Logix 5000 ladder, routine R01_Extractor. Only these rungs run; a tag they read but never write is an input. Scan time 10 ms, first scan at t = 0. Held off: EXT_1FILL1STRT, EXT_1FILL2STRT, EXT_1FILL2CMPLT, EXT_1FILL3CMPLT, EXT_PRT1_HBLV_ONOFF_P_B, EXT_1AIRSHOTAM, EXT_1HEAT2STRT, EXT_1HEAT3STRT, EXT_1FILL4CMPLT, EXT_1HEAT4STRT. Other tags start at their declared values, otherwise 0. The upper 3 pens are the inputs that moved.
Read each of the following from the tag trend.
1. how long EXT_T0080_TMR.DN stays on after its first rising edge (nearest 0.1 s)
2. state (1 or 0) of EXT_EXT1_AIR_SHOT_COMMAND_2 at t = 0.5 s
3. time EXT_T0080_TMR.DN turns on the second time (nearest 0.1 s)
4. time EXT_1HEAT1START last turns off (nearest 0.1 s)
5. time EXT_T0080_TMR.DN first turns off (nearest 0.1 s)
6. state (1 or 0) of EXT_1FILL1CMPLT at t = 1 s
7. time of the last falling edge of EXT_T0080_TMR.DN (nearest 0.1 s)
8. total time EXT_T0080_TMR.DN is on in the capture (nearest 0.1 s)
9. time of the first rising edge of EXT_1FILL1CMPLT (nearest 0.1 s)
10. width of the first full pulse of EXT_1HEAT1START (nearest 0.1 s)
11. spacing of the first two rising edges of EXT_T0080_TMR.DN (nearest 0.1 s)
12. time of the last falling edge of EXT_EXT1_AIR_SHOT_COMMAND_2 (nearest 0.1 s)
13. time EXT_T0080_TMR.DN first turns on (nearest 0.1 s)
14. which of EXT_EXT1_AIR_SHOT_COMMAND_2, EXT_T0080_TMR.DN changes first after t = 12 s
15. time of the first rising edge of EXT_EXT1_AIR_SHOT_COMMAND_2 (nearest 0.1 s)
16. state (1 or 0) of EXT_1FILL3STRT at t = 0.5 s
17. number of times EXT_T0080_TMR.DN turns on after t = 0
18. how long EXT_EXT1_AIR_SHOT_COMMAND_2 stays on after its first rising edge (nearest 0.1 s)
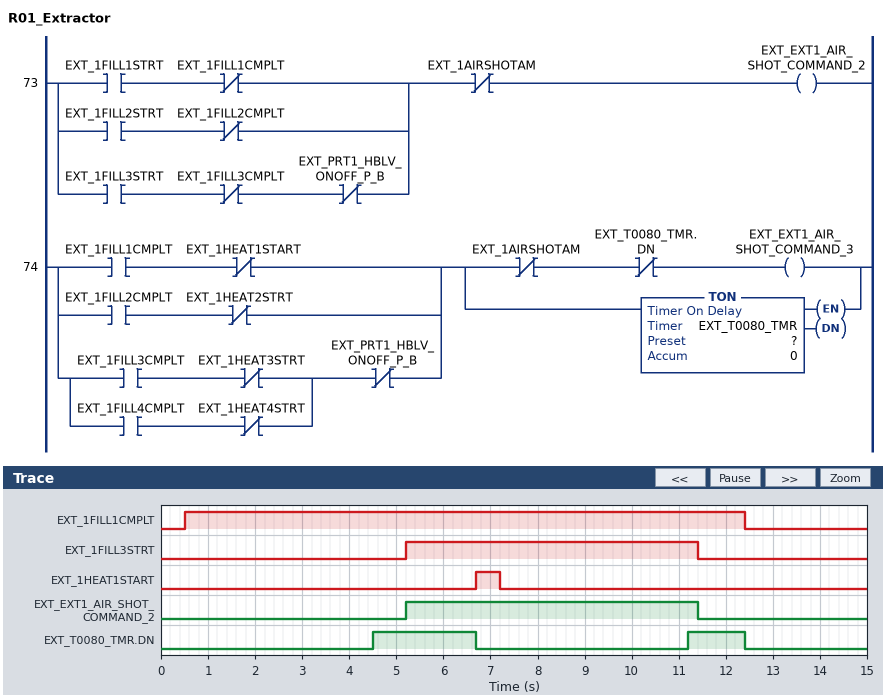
2.2 s
0
11.2 s
7.2 s
6.7 s
1
12.4 s
3.4 s
0.5 s
0.5 s
6.7 s
11.4 s
4.5 s
EXT_T0080_TMR.DN
5.2 s
0
2
6.2 s
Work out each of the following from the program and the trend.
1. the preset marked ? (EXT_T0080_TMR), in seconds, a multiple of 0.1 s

4.0 s
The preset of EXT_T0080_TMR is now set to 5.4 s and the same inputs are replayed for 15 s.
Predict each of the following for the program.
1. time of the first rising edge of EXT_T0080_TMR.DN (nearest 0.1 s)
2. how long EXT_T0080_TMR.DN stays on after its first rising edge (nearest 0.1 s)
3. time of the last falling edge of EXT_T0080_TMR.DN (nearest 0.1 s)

5.9 s
0.8 s
6.7 s
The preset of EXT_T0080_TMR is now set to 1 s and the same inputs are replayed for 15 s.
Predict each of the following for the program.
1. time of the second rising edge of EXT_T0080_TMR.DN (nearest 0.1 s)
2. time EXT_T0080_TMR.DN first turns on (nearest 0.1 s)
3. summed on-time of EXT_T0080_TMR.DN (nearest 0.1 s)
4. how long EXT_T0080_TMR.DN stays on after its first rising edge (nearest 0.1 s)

8.2 s
1.5 s
9.4 s
5.2 s
